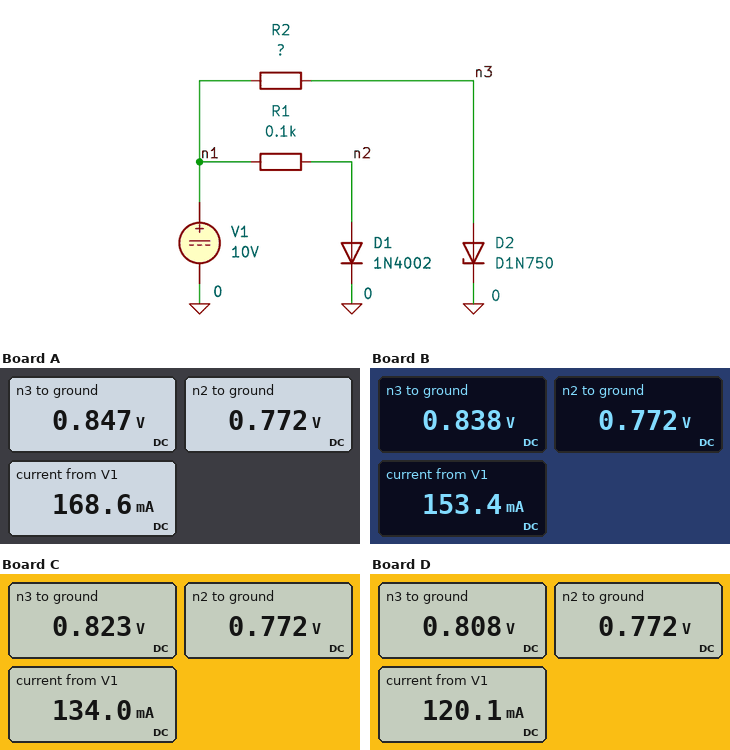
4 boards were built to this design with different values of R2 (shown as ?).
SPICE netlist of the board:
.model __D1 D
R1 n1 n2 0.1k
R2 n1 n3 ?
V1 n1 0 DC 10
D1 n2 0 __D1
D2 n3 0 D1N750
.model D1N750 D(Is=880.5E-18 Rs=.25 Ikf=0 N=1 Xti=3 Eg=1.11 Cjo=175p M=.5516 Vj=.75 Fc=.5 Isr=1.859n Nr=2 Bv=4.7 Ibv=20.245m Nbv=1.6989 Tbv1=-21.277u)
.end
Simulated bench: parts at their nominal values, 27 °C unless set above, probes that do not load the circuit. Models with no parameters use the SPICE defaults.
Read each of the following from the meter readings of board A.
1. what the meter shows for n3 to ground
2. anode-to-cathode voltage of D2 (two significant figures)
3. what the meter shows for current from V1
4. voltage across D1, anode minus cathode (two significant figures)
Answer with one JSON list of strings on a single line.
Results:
["0.847 V", "850 mV", "168.6 mA", "770 mV"]
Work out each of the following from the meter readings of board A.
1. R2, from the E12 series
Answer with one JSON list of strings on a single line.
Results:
["120 Ω"]
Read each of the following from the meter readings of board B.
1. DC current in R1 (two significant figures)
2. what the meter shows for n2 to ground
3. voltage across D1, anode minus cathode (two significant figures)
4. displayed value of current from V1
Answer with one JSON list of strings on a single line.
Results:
["92 mA", "0.772 V", "770 mV", "153.4 mA"]
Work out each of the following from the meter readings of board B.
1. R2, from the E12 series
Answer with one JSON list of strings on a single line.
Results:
["150 Ω"]
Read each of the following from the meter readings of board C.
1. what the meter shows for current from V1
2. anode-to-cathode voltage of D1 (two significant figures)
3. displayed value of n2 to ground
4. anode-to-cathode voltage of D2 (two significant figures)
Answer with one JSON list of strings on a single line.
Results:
["134.0 mA", "770 mV", "0.772 V", "820 mV"]
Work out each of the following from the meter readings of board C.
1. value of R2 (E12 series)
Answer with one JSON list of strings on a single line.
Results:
["220 Ω"]
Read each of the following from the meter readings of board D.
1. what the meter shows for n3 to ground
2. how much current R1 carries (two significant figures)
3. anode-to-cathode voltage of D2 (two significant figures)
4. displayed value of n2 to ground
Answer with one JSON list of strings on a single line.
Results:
["0.808 V", "92 mA", "810 mV", "0.772 V"]
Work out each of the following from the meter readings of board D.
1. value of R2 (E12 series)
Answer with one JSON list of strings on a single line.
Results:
["330 Ω"]
